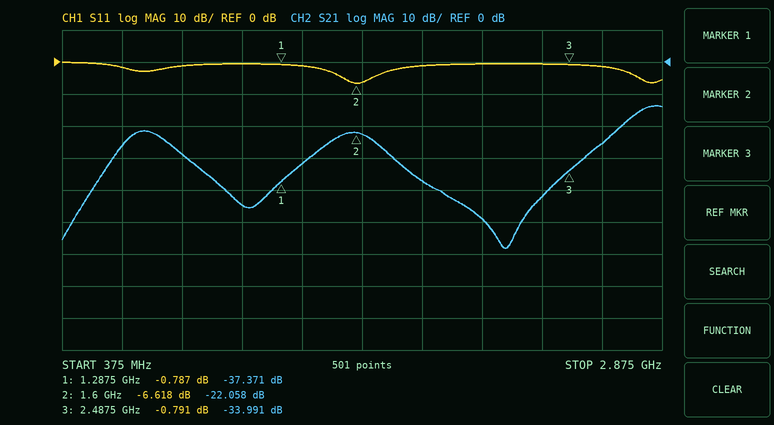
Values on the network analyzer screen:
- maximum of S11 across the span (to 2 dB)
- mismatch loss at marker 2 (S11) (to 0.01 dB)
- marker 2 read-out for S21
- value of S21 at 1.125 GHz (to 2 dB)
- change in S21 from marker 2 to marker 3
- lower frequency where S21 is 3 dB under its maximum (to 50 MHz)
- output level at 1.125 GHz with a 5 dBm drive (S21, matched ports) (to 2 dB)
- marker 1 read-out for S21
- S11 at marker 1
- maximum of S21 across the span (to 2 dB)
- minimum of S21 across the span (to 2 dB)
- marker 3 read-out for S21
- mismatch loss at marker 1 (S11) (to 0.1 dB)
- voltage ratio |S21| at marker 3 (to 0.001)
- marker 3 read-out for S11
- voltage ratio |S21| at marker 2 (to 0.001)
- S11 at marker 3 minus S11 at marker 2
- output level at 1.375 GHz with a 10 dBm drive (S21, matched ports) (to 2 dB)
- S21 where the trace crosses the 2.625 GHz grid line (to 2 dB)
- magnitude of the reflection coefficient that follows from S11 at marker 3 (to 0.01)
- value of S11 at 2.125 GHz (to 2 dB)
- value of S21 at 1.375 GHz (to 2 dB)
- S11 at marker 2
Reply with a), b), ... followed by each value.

a) 0 dB
b) 1.07 dB
c) -22.058 dB
d) -44 dB
e) -11.933 dB
f) 2.75 GHz
g) -40 dBm
h) -37.371 dB
i) -0.787 dB
j) -14 dB
k) -58 dB
l) -33.991 dB
m) 7.8 dB
n) 0.020
o) -0.791 dB
p) 0.079
q) 5.827 dB
r) -22 dBm
s) -26 dB
t) 0.91
u) 0 dB
v) -32 dB
w) -6.618 dB
